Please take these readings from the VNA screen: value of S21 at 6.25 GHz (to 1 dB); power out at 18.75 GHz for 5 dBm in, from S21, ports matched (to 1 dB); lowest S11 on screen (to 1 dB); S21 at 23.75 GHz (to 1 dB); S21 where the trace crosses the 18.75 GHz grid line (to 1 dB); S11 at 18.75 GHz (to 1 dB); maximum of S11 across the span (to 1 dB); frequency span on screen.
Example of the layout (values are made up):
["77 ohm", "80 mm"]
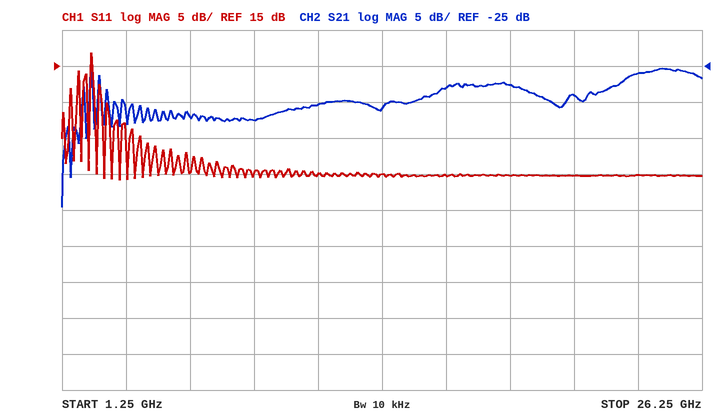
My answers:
["-32 dB", "-23 dBm", "-1 dB", "-26 dB", "-28 dB", "0 dB", "17 dB", "25 GHz"]
